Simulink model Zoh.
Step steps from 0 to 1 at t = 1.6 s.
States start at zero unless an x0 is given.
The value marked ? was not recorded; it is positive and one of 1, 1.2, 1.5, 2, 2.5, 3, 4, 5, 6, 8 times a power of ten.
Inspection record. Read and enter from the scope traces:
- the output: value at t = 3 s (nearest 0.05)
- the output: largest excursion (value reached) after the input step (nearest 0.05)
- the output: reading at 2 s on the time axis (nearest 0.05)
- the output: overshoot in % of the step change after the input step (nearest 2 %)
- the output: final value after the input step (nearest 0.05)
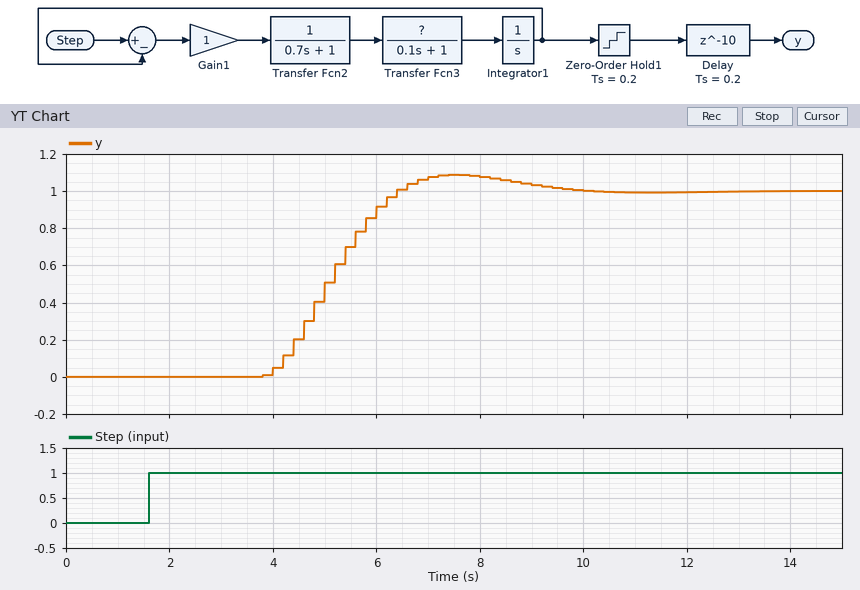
0.00
1.10
0.00
8 %
1.00
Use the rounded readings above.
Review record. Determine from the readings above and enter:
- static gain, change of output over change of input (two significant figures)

1.0
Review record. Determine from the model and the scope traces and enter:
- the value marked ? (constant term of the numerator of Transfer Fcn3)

0.8
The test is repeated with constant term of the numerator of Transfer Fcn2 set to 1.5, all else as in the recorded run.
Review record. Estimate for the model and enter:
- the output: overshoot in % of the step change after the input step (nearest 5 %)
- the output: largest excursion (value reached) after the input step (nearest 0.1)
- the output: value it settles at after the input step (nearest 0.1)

20 %
1.2
1.0
